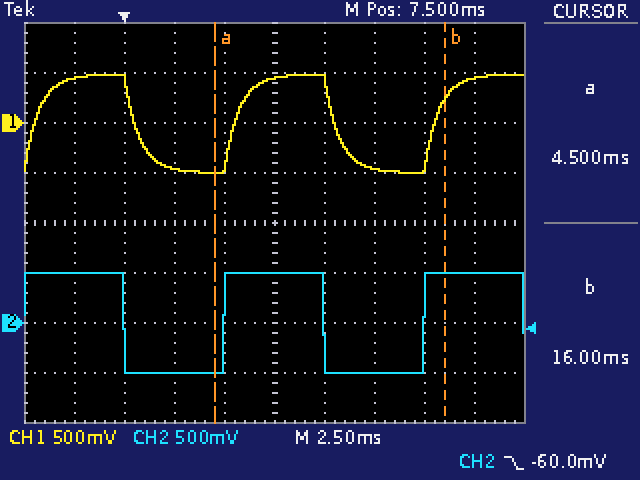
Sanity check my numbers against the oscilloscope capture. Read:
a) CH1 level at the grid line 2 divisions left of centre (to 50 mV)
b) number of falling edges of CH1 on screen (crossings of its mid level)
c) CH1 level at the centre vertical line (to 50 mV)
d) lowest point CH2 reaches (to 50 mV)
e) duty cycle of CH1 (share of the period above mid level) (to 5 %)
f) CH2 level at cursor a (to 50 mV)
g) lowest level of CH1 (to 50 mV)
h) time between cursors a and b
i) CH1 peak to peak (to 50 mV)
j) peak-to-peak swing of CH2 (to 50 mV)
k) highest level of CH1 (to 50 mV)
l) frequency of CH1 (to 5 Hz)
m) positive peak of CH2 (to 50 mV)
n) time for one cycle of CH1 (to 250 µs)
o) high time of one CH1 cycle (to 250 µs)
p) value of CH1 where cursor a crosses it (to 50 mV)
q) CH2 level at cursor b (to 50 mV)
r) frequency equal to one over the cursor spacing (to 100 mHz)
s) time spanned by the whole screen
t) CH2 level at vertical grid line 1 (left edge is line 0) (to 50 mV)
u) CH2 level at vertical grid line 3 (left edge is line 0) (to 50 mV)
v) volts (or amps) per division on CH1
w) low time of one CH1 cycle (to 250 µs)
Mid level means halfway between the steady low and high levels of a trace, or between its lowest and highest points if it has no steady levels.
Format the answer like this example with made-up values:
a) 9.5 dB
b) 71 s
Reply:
a) -450 mV
b) 2
c) 450 mV
d) -500 mV
e) 50 %
f) -500 mV
g) -500 mV
h) 11.50 ms
i) 1.00 V
j) 1.00 V
k) 500 mV
l) 100 Hz
m) 500 mV
n) 10.00 ms
o) 5.00 ms
p) -500 mV
q) 500 mV
r) 87.0 Hz
s) 25 ms
t) 500 mV
u) -500 mV
v) 500 mV
w) 5.00 ms
